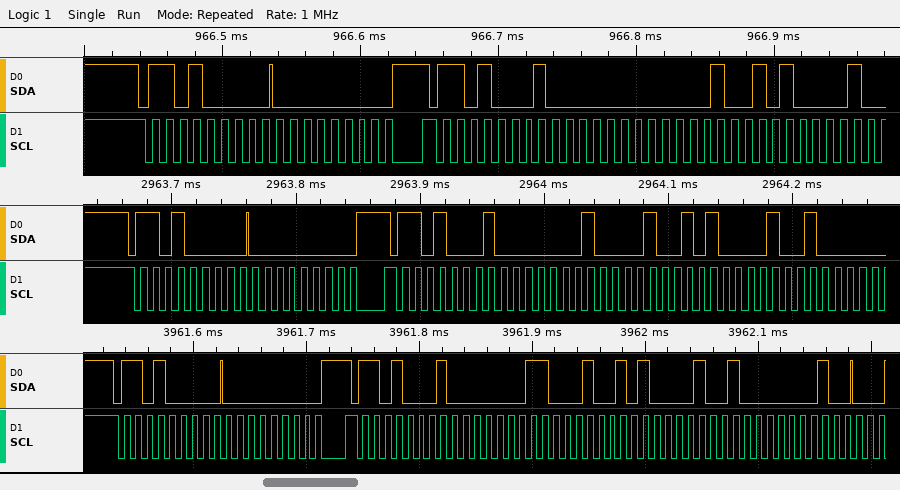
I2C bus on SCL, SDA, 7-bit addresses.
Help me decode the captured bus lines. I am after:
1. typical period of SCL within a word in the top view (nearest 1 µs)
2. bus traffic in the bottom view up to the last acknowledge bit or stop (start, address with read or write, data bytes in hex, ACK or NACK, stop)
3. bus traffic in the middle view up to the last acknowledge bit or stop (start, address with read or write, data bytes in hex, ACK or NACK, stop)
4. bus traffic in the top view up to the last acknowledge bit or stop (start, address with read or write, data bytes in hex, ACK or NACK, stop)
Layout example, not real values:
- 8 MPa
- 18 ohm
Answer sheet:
- 10 µs
- start, address 68 write ACK, 00 ACK, repeated start, address 68 read ACK, 03 ACK, 25 ACK, 12 ACK, 04 ACK
- start, address 68 write ACK, 00 ACK, repeated start, address 68 read ACK, 02 ACK, 25 ACK, 12 ACK
- start, address 68 write ACK, 00 ACK, repeated start, address 68 read ACK, 00 ACK, 25 ACK
